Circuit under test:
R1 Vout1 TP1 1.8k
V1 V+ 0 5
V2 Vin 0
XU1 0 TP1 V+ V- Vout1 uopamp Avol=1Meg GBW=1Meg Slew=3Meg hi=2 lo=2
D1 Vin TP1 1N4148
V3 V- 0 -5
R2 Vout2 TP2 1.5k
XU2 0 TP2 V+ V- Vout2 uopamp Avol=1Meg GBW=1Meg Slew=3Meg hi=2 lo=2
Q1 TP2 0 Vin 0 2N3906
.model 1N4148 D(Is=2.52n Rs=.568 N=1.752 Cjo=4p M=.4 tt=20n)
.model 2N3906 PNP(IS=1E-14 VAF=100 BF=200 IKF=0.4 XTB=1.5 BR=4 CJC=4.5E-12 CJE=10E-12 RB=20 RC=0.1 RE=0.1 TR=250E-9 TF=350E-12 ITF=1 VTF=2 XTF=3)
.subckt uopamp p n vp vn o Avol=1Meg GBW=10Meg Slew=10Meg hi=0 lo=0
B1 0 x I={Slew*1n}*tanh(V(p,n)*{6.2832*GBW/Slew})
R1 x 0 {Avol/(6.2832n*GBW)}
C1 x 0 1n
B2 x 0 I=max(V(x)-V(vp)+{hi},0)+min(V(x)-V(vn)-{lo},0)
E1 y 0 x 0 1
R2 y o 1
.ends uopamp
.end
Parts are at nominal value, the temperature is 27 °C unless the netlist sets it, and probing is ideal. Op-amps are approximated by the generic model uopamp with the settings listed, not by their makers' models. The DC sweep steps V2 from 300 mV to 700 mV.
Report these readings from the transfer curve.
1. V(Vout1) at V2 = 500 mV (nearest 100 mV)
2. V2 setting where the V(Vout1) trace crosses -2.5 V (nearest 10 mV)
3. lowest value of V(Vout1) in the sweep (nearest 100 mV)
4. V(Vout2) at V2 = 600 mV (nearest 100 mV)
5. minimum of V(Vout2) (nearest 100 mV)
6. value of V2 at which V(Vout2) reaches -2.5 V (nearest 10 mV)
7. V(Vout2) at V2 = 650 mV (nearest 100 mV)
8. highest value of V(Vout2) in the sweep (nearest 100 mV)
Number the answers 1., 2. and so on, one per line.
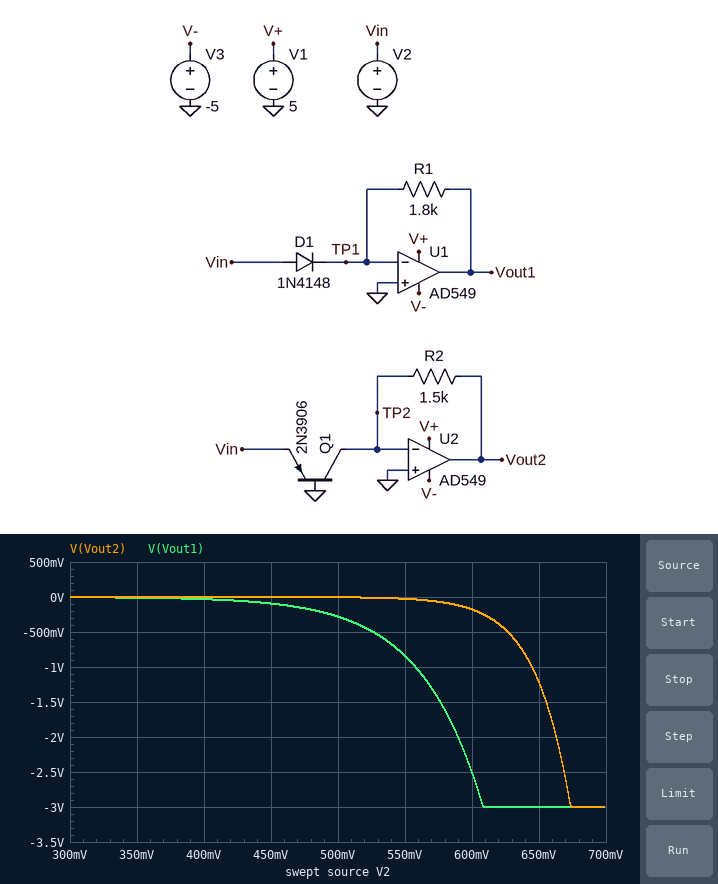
1. -300 mV
2. 600 mV
3. -3.0 V
4. -200 mV
5. -3.0 V
6. 670 mV
7. -1.2 V
8. 0 V
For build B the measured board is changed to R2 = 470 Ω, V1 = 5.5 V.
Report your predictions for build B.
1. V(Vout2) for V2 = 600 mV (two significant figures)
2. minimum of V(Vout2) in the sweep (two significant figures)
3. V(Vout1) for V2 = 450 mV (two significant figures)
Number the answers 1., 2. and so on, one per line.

1. -56 mV
2. -2.5 V
3. -93 mV
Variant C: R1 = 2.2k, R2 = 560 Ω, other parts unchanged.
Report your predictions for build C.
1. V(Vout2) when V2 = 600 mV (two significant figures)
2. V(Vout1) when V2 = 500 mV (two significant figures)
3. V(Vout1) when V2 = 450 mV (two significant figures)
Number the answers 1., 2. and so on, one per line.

1. -66 mV
2. -340 mV
3. -110 mV
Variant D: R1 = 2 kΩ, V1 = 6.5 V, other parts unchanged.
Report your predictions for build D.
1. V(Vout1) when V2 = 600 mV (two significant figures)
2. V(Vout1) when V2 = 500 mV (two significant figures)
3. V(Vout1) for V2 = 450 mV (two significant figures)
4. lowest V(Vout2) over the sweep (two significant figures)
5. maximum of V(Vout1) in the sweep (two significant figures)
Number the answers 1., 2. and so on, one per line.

1. -2.8 V
2. -310 mV
3. -100 mV
4. -3.0 V
5. -3.8 mV
